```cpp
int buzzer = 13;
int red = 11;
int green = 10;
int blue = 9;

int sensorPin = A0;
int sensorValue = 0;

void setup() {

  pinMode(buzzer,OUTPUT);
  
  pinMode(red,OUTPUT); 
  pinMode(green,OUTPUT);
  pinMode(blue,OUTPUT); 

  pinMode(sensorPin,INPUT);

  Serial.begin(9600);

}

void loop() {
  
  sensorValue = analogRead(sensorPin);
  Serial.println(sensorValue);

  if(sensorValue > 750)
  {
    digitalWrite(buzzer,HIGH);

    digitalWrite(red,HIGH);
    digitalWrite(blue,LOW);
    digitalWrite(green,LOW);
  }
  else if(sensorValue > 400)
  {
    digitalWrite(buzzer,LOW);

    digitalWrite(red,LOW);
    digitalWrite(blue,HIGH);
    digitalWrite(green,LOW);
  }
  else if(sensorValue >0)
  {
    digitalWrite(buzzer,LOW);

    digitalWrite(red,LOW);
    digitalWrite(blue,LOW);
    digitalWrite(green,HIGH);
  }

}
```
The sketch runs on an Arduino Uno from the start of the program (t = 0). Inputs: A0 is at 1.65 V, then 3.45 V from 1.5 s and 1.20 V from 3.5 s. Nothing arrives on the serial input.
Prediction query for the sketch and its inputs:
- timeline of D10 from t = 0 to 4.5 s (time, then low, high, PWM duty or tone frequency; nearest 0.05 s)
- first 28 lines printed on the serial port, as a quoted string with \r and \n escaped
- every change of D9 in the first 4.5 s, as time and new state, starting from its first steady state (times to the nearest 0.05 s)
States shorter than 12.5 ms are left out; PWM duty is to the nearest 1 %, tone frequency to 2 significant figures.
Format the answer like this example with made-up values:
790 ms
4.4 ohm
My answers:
0 s high; 1.5 s low; 3.5 s high
"337\r\n337\r\n337\r\n337\r\n337\r\n337\r\n337\r\n337\r\n337\r\n337\r\n337\r\n337\r\n337\r\n337\r\n337\r\n337\r\n337\r\n337\r\n337\r\n337\r\n337\r\n337\r\n337\r\n337\r\n337\r\n337\r\n337\r\n337\r\n"
0 s low; 1.5 s high; 3.5 s low
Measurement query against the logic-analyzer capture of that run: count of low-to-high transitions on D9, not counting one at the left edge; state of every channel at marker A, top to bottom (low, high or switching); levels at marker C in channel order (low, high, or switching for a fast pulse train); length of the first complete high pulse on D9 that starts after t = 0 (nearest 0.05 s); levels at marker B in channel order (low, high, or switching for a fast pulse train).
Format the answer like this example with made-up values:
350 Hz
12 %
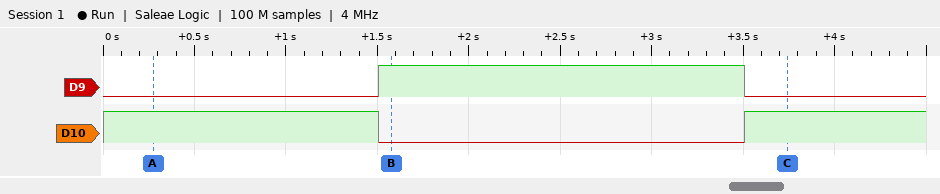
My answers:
1
D9 low, D10 high
D9 low, D10 high
2.00 s
D9 high, D10 low
